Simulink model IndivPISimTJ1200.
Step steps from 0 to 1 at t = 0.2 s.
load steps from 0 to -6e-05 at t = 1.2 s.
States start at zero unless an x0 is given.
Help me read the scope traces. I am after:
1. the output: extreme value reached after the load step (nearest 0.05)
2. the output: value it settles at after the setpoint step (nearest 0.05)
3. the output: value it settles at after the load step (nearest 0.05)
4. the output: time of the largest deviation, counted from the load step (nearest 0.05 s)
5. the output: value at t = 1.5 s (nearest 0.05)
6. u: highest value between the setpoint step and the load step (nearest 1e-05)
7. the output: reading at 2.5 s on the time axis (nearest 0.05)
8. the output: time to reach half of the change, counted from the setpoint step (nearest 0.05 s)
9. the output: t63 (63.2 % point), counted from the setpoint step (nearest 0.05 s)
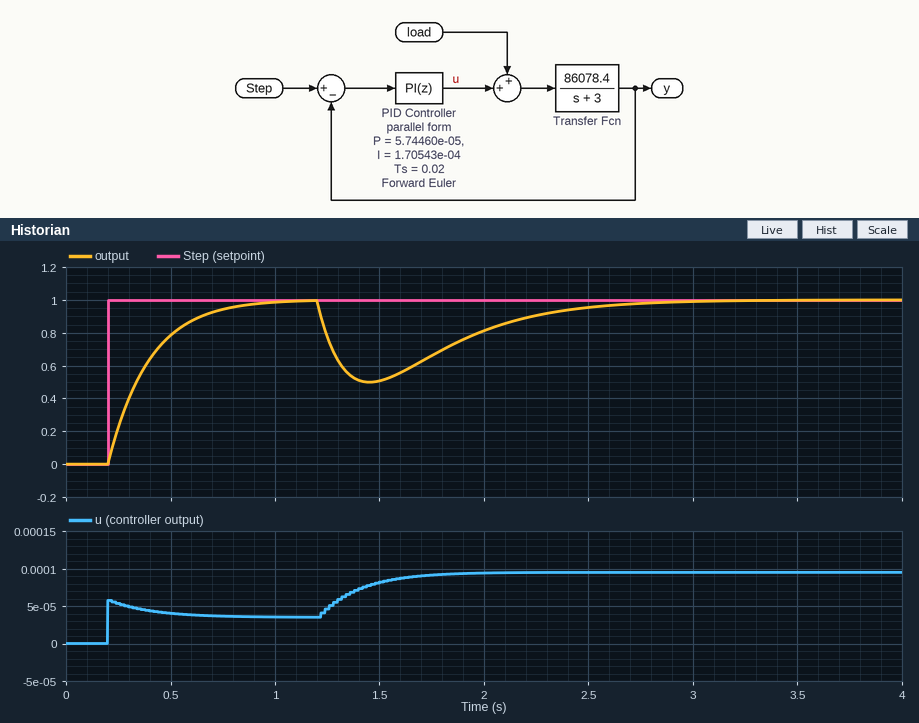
0.50
1.00
1.00
0.25 s
0.50
0.00006
0.95
0.15 s
0.20 s
